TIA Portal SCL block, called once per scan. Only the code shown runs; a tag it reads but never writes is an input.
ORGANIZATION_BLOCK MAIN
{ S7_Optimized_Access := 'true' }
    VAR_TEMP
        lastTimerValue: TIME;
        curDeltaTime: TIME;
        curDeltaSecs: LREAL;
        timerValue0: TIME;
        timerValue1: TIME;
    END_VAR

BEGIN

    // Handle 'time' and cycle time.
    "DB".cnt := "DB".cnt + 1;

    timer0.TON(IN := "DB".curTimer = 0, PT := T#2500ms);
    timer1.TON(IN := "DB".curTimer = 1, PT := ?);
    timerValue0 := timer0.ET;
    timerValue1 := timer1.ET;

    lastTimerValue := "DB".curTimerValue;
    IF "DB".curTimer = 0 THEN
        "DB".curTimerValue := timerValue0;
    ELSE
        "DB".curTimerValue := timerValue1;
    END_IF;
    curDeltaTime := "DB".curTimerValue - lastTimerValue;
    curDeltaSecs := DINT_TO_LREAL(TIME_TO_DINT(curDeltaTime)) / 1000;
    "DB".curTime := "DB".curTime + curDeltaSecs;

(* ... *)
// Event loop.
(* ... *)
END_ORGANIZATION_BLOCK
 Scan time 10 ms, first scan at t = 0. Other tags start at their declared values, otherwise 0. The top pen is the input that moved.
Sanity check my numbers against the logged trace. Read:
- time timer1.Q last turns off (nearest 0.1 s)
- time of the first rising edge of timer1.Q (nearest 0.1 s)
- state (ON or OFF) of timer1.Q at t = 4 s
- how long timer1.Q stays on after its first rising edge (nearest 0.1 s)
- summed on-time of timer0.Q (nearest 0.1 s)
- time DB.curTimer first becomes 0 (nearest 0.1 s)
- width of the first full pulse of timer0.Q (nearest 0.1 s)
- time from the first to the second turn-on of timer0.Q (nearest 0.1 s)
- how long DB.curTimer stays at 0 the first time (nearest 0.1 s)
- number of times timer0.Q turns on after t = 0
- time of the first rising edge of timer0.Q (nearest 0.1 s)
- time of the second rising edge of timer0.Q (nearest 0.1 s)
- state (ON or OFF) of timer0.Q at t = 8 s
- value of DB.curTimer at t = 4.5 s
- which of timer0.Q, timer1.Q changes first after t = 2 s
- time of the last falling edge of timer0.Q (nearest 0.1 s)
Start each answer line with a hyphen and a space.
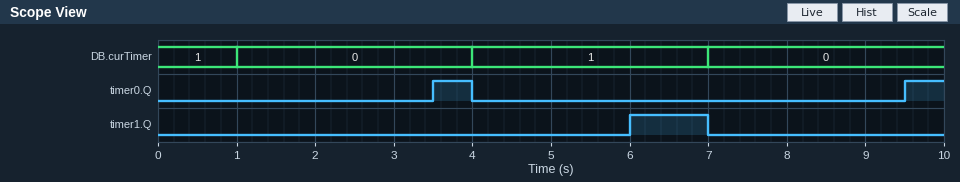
- 7.0 s
- 6.0 s
- OFF
- 1.0 s
- 1.0 s
- 1.0 s
- 0.5 s
- 6.0 s
- 3.0 s
- 2
- 3.5 s
- 9.5 s
- OFF
- 1
- timer0.Q
- 4.0 s
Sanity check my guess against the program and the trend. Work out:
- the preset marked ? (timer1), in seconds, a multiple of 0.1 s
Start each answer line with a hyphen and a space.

- 2.0 s
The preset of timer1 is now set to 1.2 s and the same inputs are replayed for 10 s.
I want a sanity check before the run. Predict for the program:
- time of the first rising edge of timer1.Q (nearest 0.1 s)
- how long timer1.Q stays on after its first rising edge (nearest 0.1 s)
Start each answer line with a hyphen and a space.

- 5.2 s
- 1.8 s
